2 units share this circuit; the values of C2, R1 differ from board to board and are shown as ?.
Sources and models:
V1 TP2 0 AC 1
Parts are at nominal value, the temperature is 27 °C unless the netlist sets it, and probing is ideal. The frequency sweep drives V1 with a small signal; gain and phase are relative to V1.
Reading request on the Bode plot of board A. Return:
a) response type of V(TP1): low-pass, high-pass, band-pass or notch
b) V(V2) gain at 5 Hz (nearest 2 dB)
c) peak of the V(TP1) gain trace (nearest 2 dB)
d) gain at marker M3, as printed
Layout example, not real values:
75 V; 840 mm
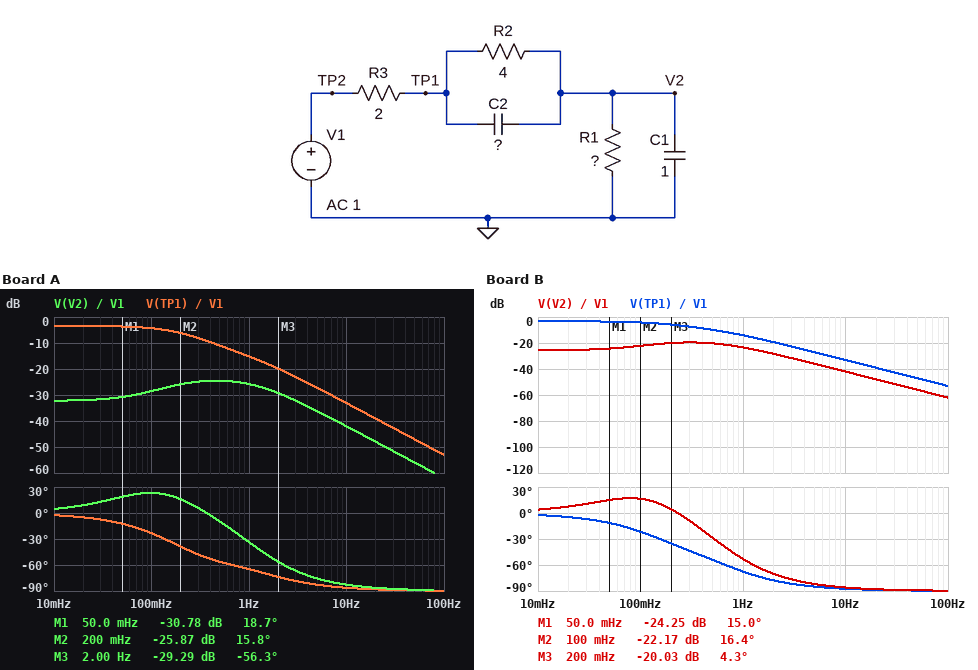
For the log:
low-pass; -36 dB; -4 dB; -29.29 dB
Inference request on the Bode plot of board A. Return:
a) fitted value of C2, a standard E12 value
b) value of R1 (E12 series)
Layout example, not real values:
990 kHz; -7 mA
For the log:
560 mF; 0.15 Ω
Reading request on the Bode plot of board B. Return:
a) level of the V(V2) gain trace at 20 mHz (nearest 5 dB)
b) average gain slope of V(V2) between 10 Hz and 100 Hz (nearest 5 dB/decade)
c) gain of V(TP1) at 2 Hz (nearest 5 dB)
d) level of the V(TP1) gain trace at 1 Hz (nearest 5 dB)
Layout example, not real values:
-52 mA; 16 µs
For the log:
-25 dB; -20 dB/decade; -20 dB; -15 dB
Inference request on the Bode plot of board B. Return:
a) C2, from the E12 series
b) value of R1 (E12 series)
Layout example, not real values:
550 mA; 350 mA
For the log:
560 mF; 0.33 Ω
